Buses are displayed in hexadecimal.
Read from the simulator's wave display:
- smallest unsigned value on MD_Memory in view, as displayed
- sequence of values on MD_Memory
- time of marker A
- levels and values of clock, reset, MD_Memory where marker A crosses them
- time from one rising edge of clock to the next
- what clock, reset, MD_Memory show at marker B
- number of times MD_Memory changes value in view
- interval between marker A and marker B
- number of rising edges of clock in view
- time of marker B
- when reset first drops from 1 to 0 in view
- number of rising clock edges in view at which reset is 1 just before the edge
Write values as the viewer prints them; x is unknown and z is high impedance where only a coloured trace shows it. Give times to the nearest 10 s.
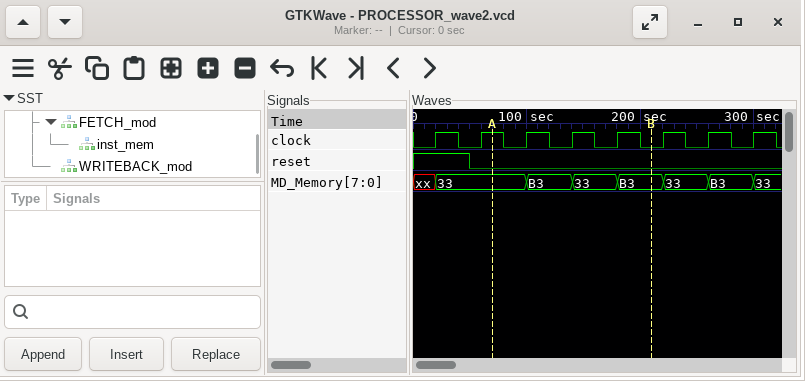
33
xx, 33, B3, 33, B3, 33, B3, 33
70 s
clock=1, reset=0, MD_Memory=33
40 s
clock=0, reset=0, MD_Memory=B3
7
140 s
8
210 s
50 s
1
